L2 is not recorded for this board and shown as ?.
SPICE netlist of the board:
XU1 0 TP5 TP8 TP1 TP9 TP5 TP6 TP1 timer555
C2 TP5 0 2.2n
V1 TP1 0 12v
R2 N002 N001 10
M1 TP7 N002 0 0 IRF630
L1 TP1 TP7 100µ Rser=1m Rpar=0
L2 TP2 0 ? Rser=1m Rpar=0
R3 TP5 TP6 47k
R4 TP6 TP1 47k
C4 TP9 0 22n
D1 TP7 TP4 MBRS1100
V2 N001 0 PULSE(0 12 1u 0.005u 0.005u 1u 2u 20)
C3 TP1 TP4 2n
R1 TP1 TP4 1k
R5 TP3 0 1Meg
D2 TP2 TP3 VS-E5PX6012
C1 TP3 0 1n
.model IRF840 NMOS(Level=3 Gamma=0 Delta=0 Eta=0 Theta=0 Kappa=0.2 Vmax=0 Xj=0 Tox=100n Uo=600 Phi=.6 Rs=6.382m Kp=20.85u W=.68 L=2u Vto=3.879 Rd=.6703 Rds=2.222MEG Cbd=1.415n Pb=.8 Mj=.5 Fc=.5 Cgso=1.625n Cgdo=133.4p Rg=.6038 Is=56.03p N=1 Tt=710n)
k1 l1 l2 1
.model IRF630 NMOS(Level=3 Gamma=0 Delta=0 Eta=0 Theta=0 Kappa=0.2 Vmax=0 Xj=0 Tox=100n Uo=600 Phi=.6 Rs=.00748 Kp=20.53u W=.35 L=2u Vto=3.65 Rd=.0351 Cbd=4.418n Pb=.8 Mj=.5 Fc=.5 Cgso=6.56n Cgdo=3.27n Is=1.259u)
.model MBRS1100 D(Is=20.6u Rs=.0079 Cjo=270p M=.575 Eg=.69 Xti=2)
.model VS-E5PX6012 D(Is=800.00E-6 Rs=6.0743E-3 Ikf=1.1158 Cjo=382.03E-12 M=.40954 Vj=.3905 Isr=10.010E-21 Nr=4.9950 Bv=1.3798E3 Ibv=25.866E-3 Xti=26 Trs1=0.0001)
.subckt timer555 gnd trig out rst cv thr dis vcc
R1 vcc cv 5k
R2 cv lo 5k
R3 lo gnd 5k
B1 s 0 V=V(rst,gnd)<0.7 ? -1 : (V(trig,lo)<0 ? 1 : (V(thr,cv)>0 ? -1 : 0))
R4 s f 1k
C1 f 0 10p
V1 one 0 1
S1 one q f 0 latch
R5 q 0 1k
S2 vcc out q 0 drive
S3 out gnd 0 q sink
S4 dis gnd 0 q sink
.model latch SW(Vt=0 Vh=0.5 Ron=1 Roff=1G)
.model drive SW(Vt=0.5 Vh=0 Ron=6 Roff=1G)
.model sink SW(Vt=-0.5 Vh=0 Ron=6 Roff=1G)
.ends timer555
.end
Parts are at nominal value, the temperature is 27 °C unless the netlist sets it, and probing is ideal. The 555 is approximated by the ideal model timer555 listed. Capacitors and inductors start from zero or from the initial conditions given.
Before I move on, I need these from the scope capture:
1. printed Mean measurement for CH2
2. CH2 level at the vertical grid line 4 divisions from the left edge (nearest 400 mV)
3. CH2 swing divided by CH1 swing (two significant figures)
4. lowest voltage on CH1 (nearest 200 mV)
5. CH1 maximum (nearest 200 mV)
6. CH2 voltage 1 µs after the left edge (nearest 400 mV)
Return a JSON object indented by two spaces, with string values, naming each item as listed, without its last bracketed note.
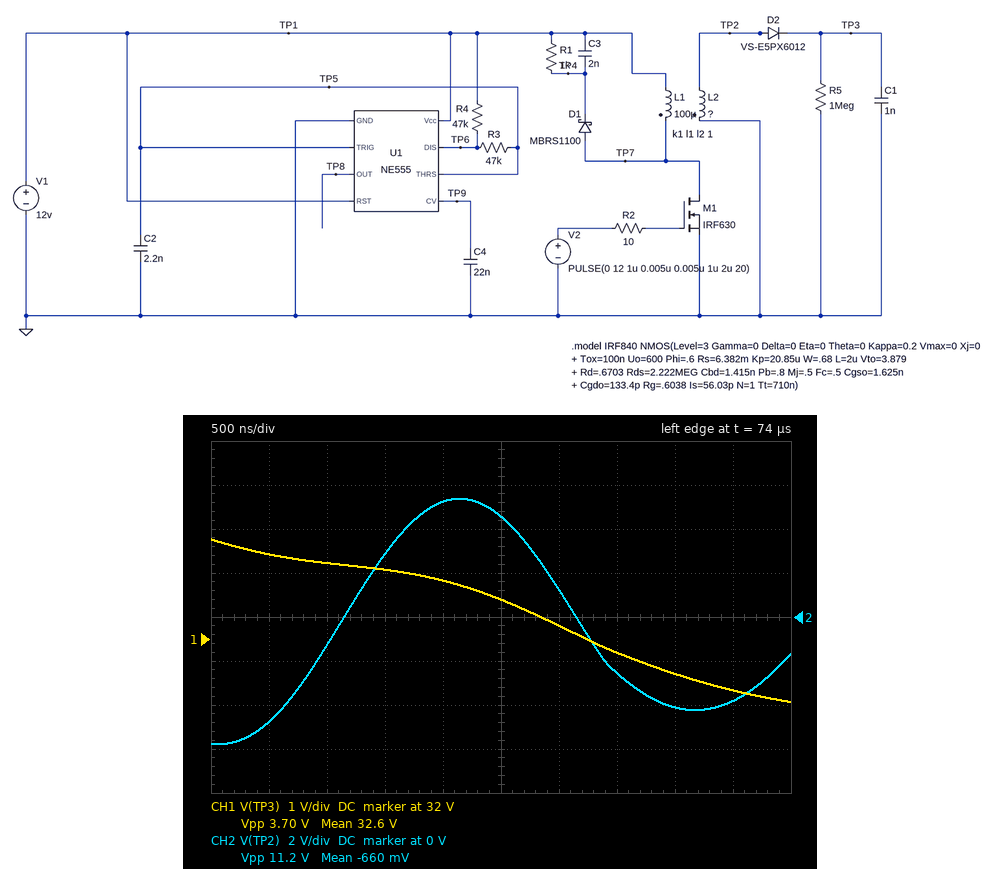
{
  "printed Mean measurement for CH2": "-660 mV",
  "CH2 level at the vertical grid line 4 divisions from the left edge": "5.2 V",
  "CH2 swing divided by CH1 swing": "3.0",
  "lowest voltage on CH1": "30.6 V",
  "CH1 maximum": "34.2 V",
  "CH2 voltage 1 µs after the left edge": "-1.2 V"
}
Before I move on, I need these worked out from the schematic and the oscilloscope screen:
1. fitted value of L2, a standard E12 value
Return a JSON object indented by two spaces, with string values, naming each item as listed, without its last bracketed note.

{
  "fitted value of L2, a standard E12 value": "2.7 mH"
}
